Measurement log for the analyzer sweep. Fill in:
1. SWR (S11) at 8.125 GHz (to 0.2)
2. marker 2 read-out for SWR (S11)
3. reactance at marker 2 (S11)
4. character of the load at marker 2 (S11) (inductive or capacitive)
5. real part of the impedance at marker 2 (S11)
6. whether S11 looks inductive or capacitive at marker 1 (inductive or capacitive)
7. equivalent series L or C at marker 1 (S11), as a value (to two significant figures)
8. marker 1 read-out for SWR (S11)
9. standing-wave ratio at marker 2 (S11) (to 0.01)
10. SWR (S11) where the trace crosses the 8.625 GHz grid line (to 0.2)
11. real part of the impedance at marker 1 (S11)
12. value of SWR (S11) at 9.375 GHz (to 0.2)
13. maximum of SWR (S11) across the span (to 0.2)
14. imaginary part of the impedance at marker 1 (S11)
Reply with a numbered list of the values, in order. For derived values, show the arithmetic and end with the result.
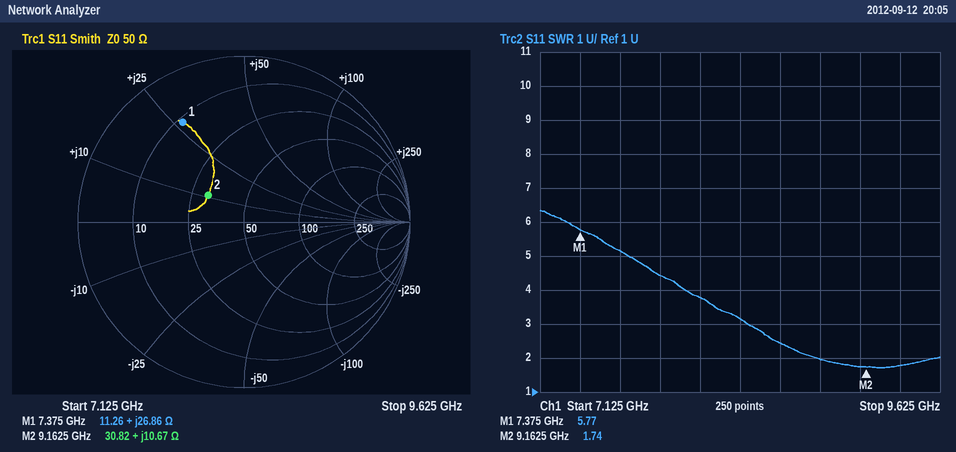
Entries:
1. 3.8
2. 1.74
3. +10.67 Ω
4. inductive
5. 30.82 Ω
6. inductive
7. L = 26.86 Ω/(2π × 7.375 GHz) ≈ 580 pH
8. 5.77
9. 1.74
10. 2.4
11. 11.26 Ω
12. 1.8
13. 6.4
14. +26.86 Ω
